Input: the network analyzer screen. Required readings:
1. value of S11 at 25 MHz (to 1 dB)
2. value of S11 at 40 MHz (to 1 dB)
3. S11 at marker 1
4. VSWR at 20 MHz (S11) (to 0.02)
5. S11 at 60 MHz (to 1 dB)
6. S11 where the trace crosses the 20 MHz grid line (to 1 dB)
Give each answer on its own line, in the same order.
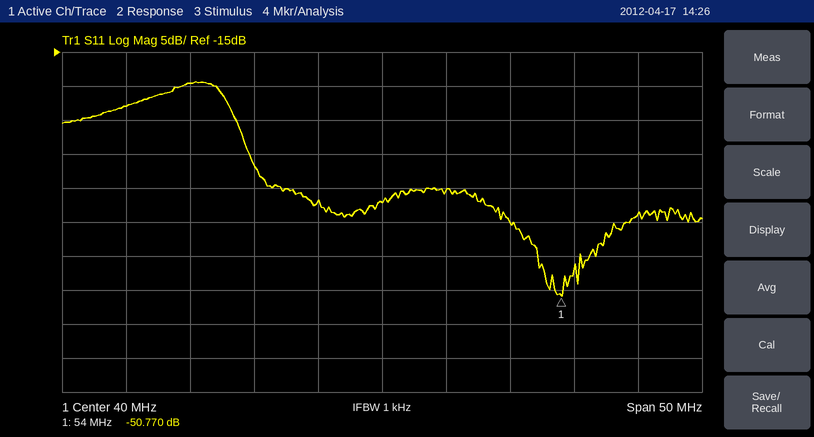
-20 dB
-37 dB
-50.770 dB
1.16
-39 dB
-23 dB
